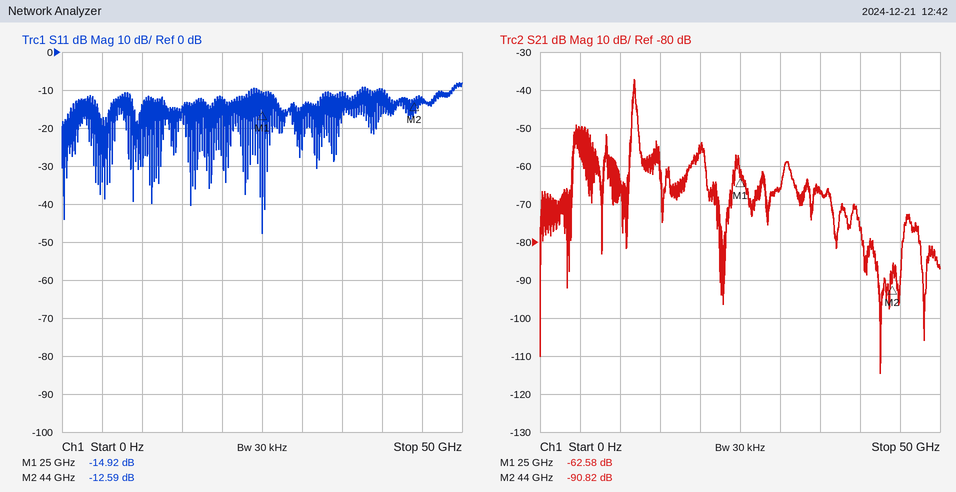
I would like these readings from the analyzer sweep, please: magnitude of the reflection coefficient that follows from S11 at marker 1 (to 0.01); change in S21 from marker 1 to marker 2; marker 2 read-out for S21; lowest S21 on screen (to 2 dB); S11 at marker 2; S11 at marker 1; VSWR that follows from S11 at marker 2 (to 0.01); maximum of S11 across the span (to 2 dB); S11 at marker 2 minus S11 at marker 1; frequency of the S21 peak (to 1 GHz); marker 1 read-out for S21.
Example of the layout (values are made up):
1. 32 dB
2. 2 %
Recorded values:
1. 0.18
2. -28.24 dB
3. -90.82 dB
4. -114 dB
5. -12.59 dB
6. -14.92 dB
7. 1.61
8. -8 dB
9. 2.33 dB
10. 12 GHz
11. -62.58 dB
